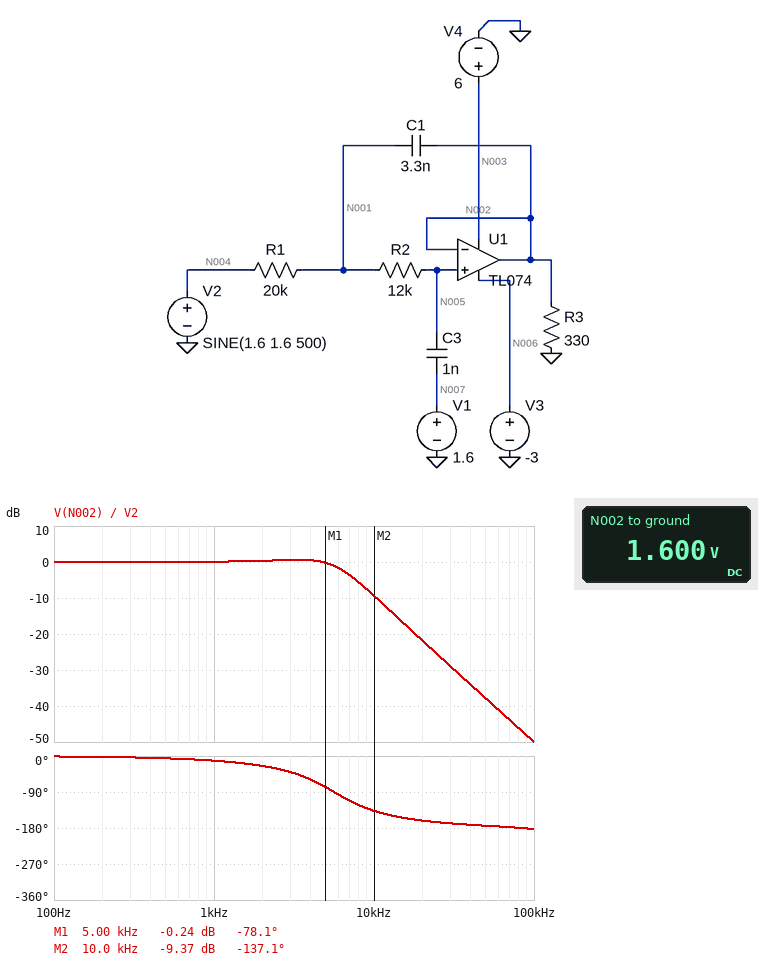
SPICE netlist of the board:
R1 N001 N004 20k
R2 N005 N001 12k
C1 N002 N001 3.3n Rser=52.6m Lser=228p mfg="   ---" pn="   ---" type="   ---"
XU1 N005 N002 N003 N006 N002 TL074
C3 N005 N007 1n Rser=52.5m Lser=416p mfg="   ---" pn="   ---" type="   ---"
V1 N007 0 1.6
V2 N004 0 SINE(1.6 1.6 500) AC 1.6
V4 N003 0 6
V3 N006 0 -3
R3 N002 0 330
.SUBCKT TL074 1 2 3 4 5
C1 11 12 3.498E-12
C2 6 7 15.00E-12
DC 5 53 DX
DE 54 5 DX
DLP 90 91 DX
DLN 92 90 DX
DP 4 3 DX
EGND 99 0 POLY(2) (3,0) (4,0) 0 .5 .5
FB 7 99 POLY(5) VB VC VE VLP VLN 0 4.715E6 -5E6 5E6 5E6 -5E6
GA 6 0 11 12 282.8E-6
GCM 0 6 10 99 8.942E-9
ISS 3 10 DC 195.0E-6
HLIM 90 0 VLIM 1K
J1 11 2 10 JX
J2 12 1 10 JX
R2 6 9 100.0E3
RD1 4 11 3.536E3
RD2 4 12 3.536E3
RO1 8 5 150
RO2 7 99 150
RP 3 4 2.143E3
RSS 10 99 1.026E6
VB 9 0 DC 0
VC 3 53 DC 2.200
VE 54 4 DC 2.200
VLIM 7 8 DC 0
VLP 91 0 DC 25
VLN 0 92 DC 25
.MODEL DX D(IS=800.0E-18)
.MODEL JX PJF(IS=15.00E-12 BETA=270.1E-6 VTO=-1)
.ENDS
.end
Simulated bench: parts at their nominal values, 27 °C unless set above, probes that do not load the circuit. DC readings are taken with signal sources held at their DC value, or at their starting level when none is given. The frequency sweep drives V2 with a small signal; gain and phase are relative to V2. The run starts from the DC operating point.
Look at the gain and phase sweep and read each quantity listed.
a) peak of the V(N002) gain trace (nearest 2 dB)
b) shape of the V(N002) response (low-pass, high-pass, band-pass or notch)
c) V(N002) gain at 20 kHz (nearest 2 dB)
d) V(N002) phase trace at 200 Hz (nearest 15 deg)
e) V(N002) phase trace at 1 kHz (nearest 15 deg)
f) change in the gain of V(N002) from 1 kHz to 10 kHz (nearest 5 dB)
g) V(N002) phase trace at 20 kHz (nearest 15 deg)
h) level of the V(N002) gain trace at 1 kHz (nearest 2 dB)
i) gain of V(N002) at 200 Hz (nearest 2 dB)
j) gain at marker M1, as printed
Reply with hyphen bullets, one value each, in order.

- 0 dB
- low-pass
- -22 dB
- 0 deg
- -15 deg
- -10 dB
- -165 deg
- 0 dB
- 0 dB
- -0.24 dB
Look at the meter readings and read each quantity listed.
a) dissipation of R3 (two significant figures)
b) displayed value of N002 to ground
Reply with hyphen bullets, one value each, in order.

- 7.8 mW
- 1.600 V
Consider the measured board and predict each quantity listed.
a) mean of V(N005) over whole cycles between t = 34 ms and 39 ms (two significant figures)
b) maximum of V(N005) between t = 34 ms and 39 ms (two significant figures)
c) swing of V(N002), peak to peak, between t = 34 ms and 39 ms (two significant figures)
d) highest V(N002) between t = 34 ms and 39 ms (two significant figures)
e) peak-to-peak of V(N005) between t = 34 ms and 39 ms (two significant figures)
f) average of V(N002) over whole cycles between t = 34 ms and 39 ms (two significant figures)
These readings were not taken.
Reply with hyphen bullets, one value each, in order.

- 1.6 V
- 3.2 V
- 3.2 V
- 3.2 V
- 3.2 V
- 1.6 V
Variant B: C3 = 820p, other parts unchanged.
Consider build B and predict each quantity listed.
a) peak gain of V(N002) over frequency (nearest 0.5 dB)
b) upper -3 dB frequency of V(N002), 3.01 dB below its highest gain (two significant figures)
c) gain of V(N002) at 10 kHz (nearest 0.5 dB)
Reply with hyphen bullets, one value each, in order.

- 1.0 dB
- 7.2 kHz
- -7.0 dB
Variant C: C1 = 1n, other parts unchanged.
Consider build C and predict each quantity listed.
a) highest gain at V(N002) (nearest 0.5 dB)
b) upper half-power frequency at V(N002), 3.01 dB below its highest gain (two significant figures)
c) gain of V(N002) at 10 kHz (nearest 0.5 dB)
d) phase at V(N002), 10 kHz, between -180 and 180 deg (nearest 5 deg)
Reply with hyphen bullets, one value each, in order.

- 0 dB
- 6.3 kHz
- -6.0 dB
- -90 deg
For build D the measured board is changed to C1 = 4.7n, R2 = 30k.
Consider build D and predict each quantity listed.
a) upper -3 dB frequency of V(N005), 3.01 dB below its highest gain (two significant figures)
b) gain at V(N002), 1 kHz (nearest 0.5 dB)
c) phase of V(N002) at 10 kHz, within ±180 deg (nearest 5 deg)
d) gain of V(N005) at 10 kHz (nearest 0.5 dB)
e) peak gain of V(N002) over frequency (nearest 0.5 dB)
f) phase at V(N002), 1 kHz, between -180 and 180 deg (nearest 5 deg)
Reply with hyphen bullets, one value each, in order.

- 3.5 kHz
- 0.5 dB
- -165 deg
- -20.5 dB
- 1.5 dB
- -20 deg
